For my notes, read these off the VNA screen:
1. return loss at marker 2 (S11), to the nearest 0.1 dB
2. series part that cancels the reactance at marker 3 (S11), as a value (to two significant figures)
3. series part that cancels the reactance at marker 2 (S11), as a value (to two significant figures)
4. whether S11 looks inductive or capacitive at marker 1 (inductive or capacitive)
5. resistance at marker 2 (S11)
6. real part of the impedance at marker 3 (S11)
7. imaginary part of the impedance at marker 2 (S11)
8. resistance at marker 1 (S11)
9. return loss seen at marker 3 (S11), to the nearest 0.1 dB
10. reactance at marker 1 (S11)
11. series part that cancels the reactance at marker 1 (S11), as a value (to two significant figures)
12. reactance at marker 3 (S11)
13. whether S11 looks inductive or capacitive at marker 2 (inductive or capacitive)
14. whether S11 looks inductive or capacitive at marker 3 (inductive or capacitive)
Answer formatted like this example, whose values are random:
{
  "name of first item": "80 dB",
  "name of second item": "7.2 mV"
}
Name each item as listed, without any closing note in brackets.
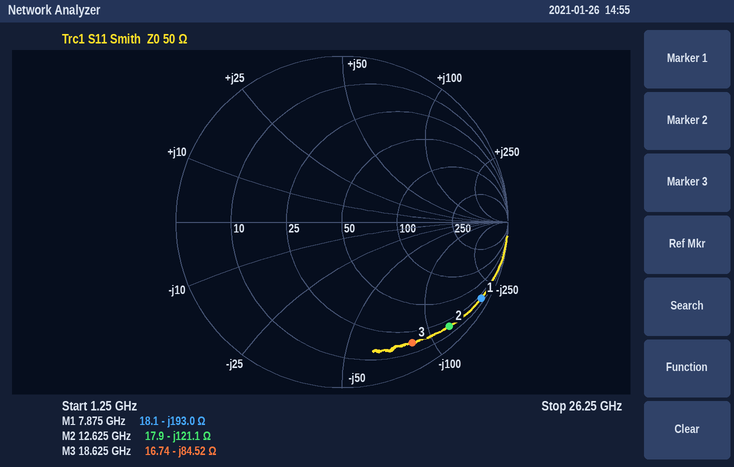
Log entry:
{
  "return loss at marker 2 (S11), to the nearest 0.1 dB": "0.9 dB",
  "series part that cancels the reactance at marker 3 (S11), as a value": "720 pH",
  "series part that cancels the reactance at marker 2 (S11), as a value": "1.5 nH",
  "whether S11 looks inductive or capacitive at marker 1": "capacitive",
  "resistance at marker 2": "17.9 Ω",
  "real part of the impedance at marker 3": "16.74 Ω",
  "imaginary part of the impedance at marker 2": "-121.1 Ω",
  "resistance at marker 1": "18.1 Ω",
  "return loss seen at marker 3 (S11), to the nearest 0.1 dB": "1.5 dB",
  "reactance at marker 1": "-193.0 Ω",
  "series part that cancels the reactance at marker 1 (S11), as a value": "3.9 nH",
  "reactance at marker 3": "-84.52 Ω",
  "whether S11 looks inductive or capacitive at marker 2": "capacitive",
  "whether S11 looks inductive or capacitive at marker 3": "capacitive"
}
